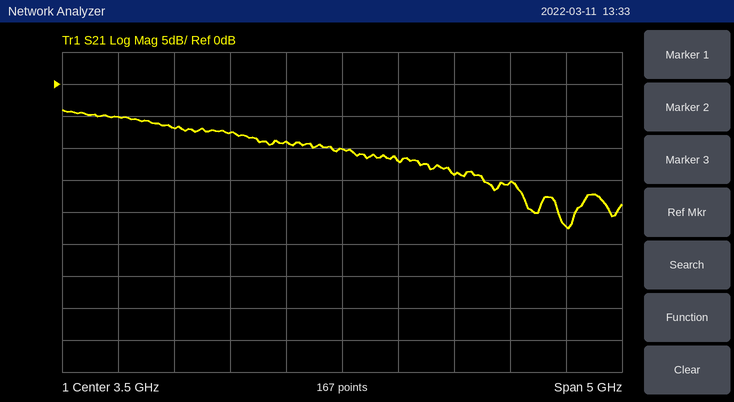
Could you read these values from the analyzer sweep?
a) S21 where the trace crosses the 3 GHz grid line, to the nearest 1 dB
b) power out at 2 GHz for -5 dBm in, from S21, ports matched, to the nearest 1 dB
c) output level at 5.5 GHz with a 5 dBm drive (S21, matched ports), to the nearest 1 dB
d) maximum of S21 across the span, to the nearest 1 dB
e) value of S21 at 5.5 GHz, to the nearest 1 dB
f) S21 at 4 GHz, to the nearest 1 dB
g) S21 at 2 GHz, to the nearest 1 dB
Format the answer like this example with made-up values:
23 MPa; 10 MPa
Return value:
-9 dB; -12 dBm; -17 dBm; -4 dB; -22 dB; -12 dB; -7 dB
